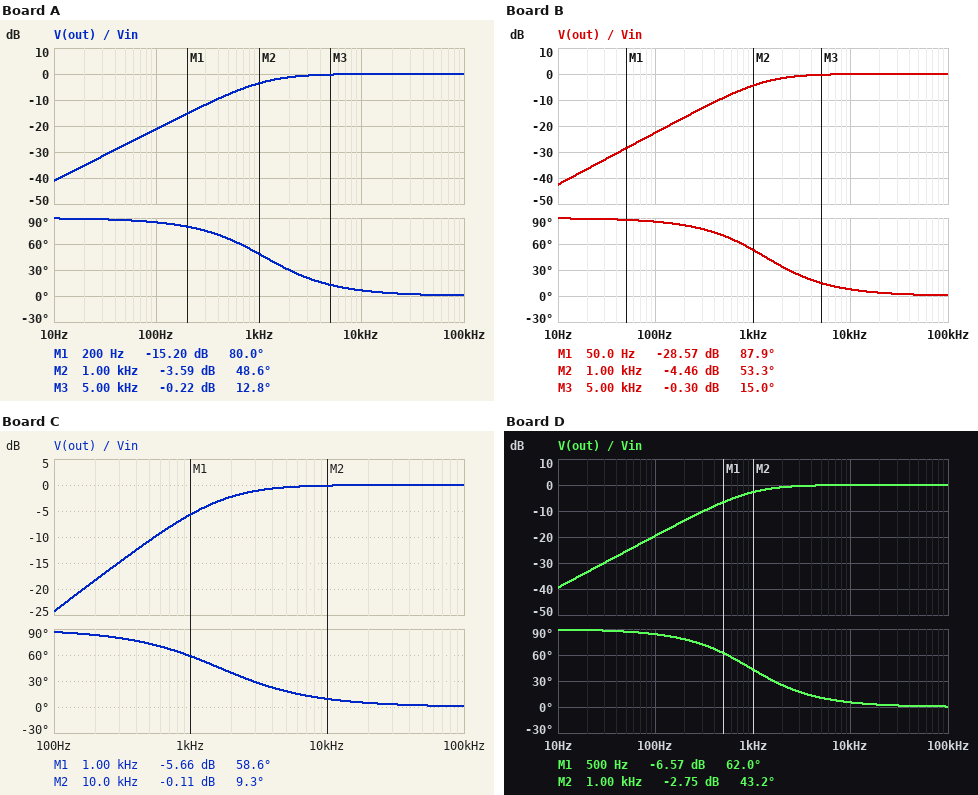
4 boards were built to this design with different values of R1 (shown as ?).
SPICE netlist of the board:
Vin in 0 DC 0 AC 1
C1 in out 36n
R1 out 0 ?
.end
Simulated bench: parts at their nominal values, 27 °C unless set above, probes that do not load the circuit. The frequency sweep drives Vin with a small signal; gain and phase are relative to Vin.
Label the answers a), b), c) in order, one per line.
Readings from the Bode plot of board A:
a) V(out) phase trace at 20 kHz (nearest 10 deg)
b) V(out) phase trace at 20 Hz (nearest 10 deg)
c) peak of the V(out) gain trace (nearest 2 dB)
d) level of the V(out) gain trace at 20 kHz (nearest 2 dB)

a) 0 deg
b) 90 deg
c) 0 dB
d) 0 dB
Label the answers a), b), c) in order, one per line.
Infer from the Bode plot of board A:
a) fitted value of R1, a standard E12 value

a) 3.9 kΩ
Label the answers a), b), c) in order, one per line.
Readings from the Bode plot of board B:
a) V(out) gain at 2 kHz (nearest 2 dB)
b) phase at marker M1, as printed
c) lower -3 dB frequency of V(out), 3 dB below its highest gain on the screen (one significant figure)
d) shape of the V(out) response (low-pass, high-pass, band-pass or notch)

a) -2 dB
b) 87.9 deg
c) 1 kHz
d) high-pass
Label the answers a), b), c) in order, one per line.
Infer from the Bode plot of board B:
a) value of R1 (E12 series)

a) 3.3 kΩ
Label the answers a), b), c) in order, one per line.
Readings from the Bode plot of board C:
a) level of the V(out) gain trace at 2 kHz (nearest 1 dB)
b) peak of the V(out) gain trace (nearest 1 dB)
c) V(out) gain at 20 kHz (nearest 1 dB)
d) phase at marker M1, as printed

a) -2 dB
b) 0 dB
c) 0 dB
d) 58.6 deg
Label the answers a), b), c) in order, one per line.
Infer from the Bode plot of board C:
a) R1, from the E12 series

a) 2.7 kΩ
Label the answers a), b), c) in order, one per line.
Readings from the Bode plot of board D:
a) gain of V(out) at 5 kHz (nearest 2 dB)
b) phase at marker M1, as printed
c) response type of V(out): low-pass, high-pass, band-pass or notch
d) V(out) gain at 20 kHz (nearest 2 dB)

a) 0 dB
b) 62.0 deg
c) high-pass
d) 0 dB
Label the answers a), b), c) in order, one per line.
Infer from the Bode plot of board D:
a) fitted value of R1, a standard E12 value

a) 4.7 kΩ
